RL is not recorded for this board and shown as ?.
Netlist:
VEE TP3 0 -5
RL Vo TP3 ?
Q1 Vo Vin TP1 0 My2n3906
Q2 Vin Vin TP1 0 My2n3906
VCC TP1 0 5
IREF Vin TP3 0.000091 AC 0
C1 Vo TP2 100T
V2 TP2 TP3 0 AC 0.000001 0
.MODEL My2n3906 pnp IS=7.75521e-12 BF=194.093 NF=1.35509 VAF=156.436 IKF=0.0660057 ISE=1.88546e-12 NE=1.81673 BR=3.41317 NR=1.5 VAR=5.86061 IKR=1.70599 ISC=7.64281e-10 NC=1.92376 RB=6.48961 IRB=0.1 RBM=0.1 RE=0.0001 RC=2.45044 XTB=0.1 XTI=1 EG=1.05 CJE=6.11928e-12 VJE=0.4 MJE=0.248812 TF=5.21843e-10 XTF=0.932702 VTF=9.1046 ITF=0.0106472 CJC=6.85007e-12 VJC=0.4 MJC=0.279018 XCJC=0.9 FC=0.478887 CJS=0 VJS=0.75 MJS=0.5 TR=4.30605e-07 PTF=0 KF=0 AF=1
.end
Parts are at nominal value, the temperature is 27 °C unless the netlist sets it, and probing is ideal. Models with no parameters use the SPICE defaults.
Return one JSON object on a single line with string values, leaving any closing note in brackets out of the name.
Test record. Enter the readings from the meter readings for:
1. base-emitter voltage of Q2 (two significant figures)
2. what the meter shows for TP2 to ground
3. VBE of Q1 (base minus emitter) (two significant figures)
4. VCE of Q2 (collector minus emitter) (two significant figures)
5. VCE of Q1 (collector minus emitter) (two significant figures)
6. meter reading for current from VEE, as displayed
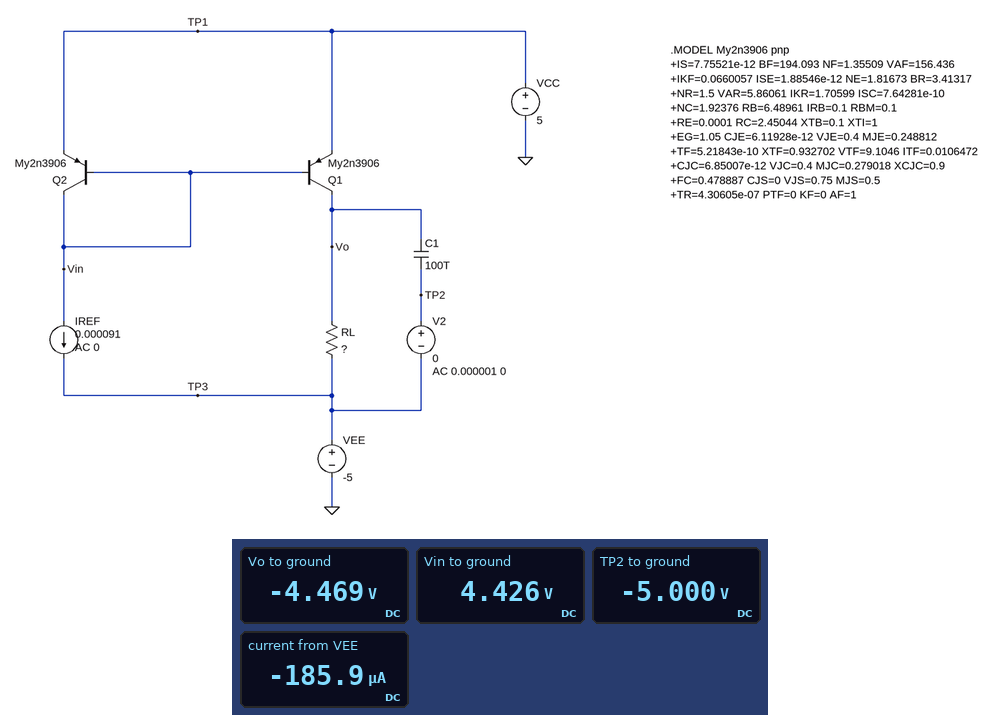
{"base-emitter voltage of Q2": "-570 mV", "what the meter shows for TP2 to ground": "-5.000 V", "VBE of Q1 (base minus emitter)": "-570 mV", "VCE of Q2 (collector minus emitter)": "-570 mV", "VCE of Q1 (collector minus emitter)": "-9.5 V", "meter reading for current from VEE, as displayed": "-185.9 µA"}
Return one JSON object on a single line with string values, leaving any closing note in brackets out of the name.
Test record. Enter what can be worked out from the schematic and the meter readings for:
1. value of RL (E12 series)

{"value of RL": "5.6 kΩ"}
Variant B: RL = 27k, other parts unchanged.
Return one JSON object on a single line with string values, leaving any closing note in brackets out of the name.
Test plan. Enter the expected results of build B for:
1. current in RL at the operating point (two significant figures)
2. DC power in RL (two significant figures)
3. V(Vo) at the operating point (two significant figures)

{"current in RL at the operating point": "94 µA", "DC power in RL": "240 µW", "V(Vo) at the operating point": "-2.5 V"}
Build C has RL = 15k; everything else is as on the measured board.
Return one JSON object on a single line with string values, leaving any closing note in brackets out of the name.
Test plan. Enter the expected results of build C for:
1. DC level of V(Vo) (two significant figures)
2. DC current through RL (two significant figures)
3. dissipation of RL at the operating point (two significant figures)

{"DC level of V(Vo)": "-3.6 V", "DC current through RL": "94 µA", "dissipation of RL at the operating point": "130 µW"}
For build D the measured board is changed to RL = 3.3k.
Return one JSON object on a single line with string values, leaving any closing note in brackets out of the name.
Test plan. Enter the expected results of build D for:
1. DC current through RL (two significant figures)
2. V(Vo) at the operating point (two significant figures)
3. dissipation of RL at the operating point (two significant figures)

{"DC current through RL": "95 µA", "V(Vo) at the operating point": "-4.7 V", "dissipation of RL at the operating point": "30 µW"}
